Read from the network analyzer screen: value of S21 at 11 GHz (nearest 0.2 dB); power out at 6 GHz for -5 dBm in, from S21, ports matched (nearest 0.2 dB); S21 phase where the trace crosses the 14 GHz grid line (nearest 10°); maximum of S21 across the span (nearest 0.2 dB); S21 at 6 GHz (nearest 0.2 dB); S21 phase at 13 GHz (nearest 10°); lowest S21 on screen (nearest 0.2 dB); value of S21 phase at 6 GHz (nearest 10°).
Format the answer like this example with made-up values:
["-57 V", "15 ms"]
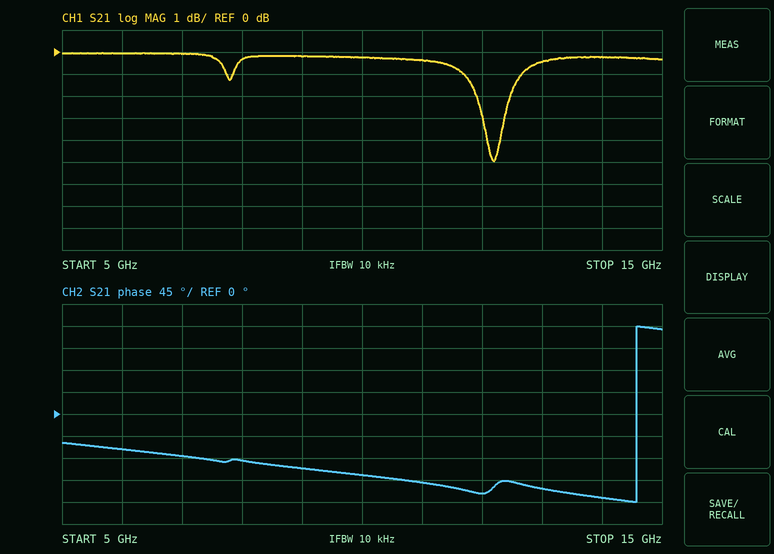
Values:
["-0.4 dB", "-5.0 dBm", "-170°", "0.0 dB", "0.0 dB", "-150°", "-5.0 dB", "-70°"]
